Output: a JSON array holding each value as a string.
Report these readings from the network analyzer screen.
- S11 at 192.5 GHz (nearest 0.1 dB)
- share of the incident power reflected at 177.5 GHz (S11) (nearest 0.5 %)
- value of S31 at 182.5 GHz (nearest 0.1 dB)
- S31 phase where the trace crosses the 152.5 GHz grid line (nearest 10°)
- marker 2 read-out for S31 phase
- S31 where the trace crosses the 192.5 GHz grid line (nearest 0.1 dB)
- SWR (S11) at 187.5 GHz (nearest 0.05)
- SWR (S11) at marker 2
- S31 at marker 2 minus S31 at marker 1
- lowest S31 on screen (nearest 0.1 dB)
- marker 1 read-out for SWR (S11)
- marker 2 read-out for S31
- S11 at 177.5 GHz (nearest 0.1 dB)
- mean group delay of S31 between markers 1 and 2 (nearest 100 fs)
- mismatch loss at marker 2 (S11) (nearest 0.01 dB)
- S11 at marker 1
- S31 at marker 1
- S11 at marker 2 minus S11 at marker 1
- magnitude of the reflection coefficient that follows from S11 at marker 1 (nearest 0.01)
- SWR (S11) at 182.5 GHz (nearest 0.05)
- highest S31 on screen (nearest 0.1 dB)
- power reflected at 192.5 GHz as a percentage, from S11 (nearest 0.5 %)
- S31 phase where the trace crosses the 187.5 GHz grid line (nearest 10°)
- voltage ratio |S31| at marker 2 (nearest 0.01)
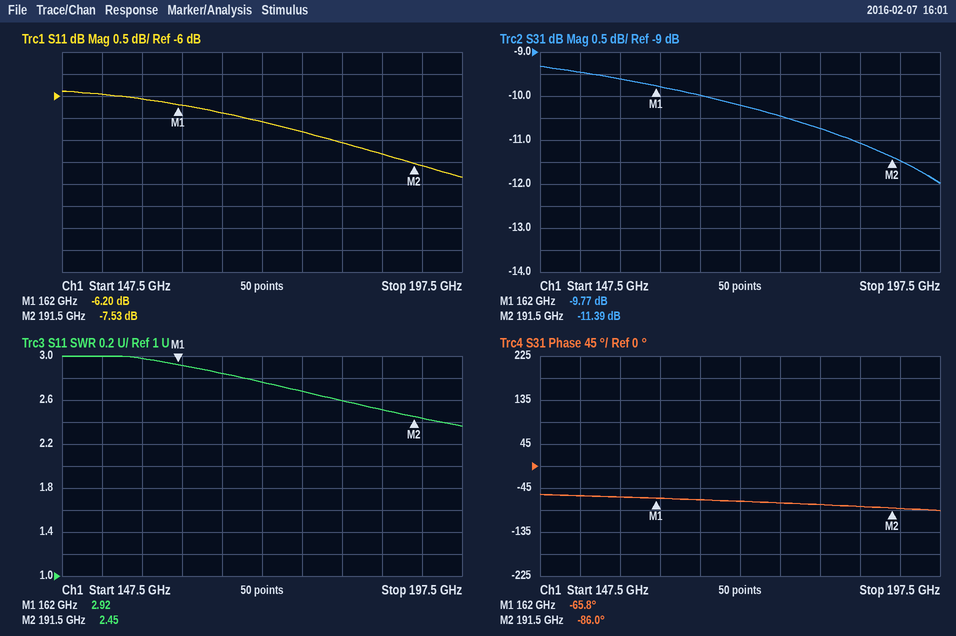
["-7.6 dB", "21.0 %", "-10.7 dB", "-60°", "-86.0°", "-11.5 dB", "2.50", "2.45", "-1.62 dB", "-12.0 dB", "2.92", "-11.39 dB", "-6.8 dB", "1.9 ps", "0.84 dB", "-6.20 dB", "-9.77 dB", "-1.33 dB", "0.49", "2.60", "-9.3 dB", "17.5 %", "-80°", "0.27"]
